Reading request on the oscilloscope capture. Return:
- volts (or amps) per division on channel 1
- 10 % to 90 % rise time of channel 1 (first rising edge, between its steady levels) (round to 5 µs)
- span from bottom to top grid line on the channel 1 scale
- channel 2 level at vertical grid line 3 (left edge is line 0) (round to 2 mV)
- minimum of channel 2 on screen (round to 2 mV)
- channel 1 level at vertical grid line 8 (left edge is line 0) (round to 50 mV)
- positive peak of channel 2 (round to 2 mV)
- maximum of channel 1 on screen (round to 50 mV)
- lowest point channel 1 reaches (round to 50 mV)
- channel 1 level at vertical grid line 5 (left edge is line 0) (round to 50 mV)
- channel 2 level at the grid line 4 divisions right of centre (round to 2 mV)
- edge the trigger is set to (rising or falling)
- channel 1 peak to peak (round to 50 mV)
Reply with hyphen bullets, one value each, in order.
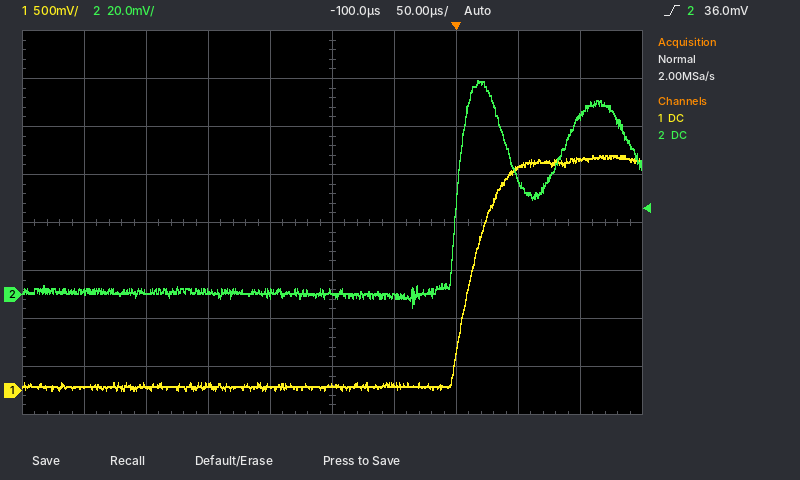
- 500 mV
- 40 µs
- 4 V
- 2 mV
- -6 mV
- 2.30 V
- 90 mV
- 2.45 V
- 0 mV
- 50 mV
- 74 mV
- rising
- 2.45 V
